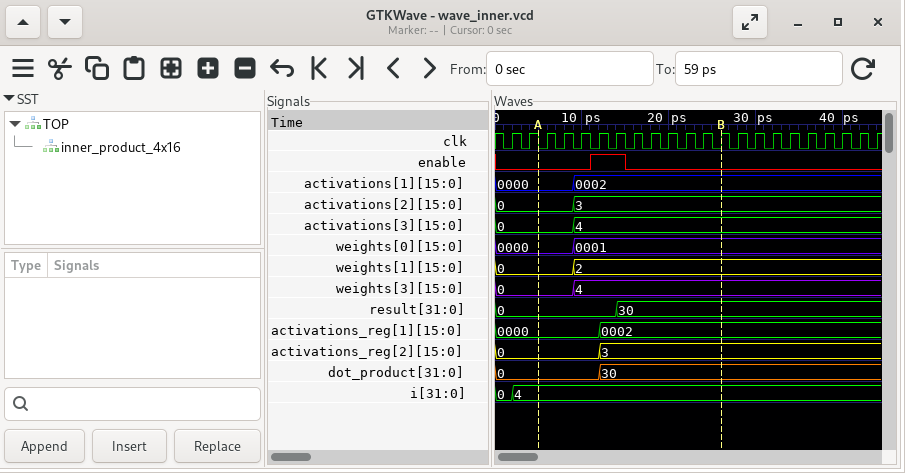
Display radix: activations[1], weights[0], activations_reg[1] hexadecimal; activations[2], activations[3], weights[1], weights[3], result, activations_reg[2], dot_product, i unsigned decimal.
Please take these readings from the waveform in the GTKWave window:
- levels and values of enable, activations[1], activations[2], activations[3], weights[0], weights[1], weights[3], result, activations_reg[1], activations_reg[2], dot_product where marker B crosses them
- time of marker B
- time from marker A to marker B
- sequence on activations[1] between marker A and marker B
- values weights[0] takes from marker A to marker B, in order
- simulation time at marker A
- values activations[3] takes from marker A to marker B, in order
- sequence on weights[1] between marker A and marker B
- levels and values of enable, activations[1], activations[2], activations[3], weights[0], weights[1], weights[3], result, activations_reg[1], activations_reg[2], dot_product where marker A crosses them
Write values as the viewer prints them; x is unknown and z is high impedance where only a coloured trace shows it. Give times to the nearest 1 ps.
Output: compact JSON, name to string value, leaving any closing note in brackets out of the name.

{"levels and values of enable, activations[1], activations[2], activations[3], weights[0], weights[1], weights[3], result, activations_reg[1], activations_reg[2], dot_product where marker B crosses them": "enable=0, activations[1]=0002, activations[2]=3, activations[3]=4, weights[0]=0001, weights[1]=2, weights[3]=4, result=30, activations_reg[1]=0002, activations_reg[2]=3, dot_product=30", "time of marker B": "26 ps", "time from marker A to marker B": "21 ps", "sequence on activations[1] between marker A and marker B": "0000, 0002", "values weights[0] takes from marker A to marker B, in order": "0000, 0001", "simulation time at marker A": "5 ps", "values activations[3] takes from marker A to marker B, in order": "0, 4", "sequence on weights[1] between marker A and marker B": "0, 2", "levels and values of enable, activations[1], activations[2], activations[3], weights[0], weights[1], weights[3], result, activations_reg[1], activations_reg[2], dot_product where marker A crosses them": "enable=0, activations[1]=0000, activations[2]=0, activations[3]=0, weights[0]=0000, weights[1]=0, weights[3]=0, result=0, activations_reg[1]=0000, activations_reg[2]=0, dot_product=0"}
